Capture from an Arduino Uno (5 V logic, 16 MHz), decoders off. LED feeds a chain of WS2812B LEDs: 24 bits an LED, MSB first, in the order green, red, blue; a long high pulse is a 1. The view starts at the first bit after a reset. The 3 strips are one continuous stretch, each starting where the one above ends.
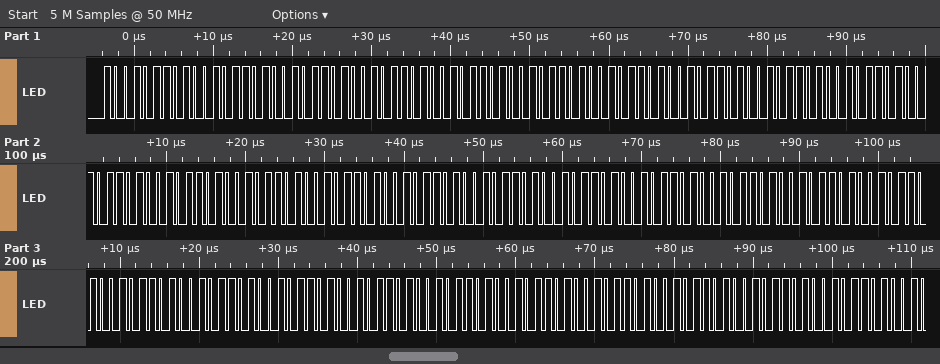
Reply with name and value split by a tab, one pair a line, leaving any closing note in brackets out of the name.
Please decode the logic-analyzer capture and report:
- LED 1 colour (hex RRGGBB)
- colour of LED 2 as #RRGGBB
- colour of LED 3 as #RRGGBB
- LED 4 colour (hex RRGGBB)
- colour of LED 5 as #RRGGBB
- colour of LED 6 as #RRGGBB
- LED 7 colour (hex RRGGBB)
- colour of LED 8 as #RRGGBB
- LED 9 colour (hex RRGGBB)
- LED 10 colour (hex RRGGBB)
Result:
LED 1 colour	#969696
colour of LED 2 as #RRGGBB	#969696
colour of LED 3 as #RRGGBB	#969696
LED 4 colour	#969696
colour of LED 5 as #RRGGBB	#969696
colour of LED 6 as #RRGGBB	#969696
LED 7 colour	#969696
colour of LED 8 as #RRGGBB	#969696
LED 9 colour	#969696
LED 10 colour	#969696
